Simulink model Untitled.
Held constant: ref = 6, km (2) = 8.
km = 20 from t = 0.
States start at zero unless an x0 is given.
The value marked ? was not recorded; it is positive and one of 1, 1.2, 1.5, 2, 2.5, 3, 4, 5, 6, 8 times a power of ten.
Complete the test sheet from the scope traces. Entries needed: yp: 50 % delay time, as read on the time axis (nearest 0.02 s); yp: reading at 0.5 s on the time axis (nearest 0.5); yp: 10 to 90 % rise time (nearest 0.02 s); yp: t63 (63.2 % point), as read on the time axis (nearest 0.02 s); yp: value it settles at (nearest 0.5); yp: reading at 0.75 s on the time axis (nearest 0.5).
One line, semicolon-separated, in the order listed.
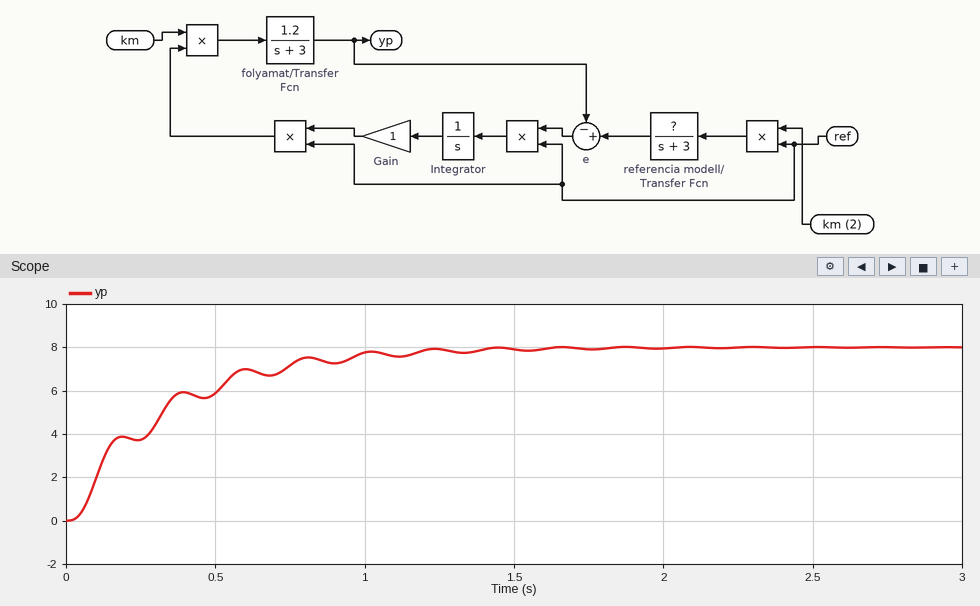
0.28 s; 6.0; 0.68 s; 0.32 s; 8.0; 7.0
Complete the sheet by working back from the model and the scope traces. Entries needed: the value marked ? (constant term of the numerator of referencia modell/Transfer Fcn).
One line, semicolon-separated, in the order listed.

0.5
